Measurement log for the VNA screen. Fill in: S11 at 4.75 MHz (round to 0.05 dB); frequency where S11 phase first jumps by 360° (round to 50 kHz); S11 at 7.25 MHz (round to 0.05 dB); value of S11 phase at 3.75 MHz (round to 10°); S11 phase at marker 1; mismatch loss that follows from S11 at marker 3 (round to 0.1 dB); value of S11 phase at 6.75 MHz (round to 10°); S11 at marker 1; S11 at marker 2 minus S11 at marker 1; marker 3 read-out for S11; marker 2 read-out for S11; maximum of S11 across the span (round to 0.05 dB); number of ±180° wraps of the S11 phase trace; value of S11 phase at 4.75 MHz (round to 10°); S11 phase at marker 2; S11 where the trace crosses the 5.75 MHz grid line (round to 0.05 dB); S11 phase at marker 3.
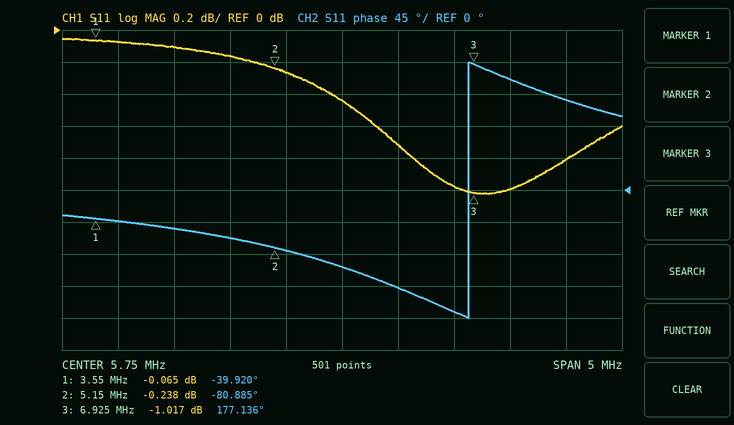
-0.15 dB
6.90 MHz
-1.00 dB
-40°
-39.920°
6.8 dB
-170°
-0.065 dB
-0.173 dB
-1.017 dB
-0.238 dB
-0.05 dB
1
-70°
-80.885°
-0.45 dB
177.136°
